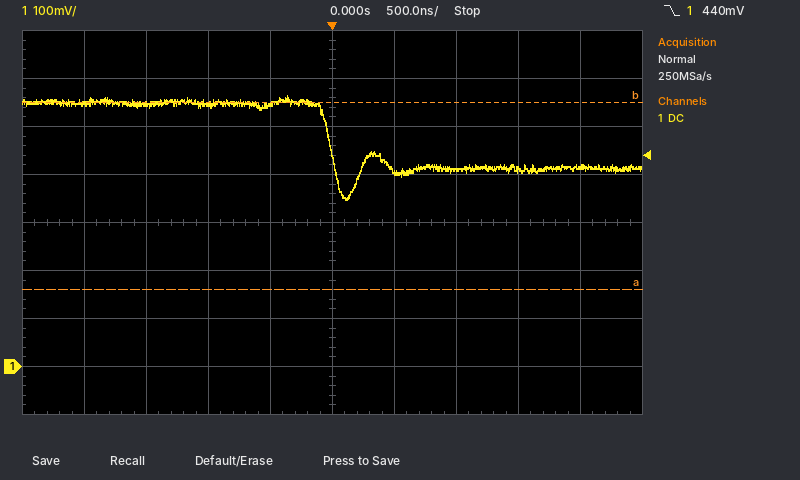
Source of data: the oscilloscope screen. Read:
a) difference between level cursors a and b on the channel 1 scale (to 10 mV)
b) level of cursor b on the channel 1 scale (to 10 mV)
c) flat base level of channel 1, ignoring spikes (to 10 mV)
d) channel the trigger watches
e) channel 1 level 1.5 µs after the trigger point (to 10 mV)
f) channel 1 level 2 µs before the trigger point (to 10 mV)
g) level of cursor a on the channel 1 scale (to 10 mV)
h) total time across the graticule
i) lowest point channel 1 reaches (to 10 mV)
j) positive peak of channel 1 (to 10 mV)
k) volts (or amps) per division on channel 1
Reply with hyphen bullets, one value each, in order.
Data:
- 390 mV
- 550 mV
- 410 mV
- channel 1
- 410 mV
- 550 mV
- 160 mV
- 5 µs
- 350 mV
- 560 mV
- 100 mV
